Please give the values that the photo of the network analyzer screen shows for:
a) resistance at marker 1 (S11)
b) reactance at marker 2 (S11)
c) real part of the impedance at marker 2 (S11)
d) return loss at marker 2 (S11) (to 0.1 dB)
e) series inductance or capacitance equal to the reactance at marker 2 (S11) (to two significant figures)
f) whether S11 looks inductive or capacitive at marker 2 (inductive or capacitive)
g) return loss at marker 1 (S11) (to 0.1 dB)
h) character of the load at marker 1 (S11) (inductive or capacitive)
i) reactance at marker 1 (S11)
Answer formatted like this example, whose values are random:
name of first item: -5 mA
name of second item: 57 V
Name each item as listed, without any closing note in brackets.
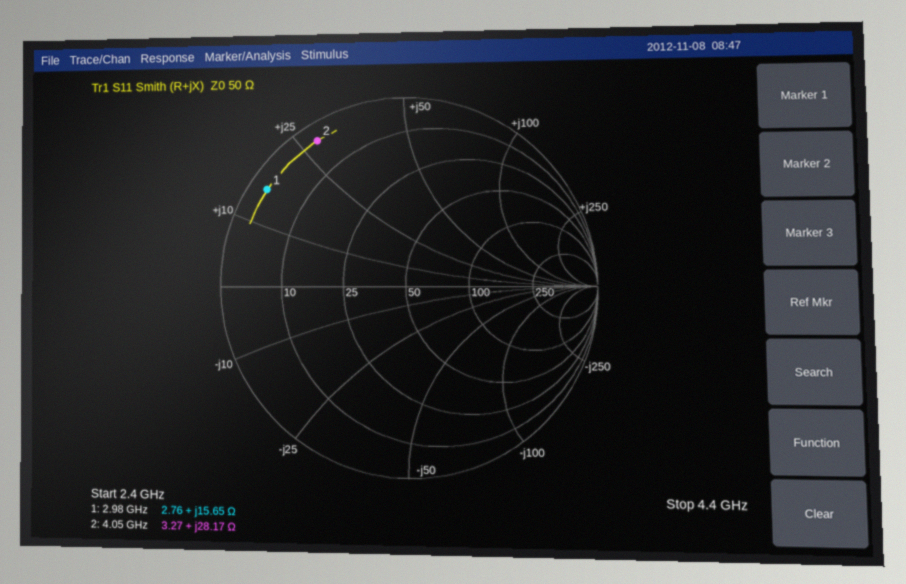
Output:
resistance at marker 1: 2.76 Ω
reactance at marker 2: +28.17 Ω
real part of the impedance at marker 2: 3.27 Ω
return loss at marker 2 (S11): 0.9 dB
series inductance or capacitance equal to the reactance at marker 2 (S11): 1.1 nH
whether S11 looks inductive or capacitive at marker 2: inductive
return loss at marker 1 (S11): 0.9 dB
character of the load at marker 1 (S11): inductive
reactance at marker 1: +15.65 Ω
